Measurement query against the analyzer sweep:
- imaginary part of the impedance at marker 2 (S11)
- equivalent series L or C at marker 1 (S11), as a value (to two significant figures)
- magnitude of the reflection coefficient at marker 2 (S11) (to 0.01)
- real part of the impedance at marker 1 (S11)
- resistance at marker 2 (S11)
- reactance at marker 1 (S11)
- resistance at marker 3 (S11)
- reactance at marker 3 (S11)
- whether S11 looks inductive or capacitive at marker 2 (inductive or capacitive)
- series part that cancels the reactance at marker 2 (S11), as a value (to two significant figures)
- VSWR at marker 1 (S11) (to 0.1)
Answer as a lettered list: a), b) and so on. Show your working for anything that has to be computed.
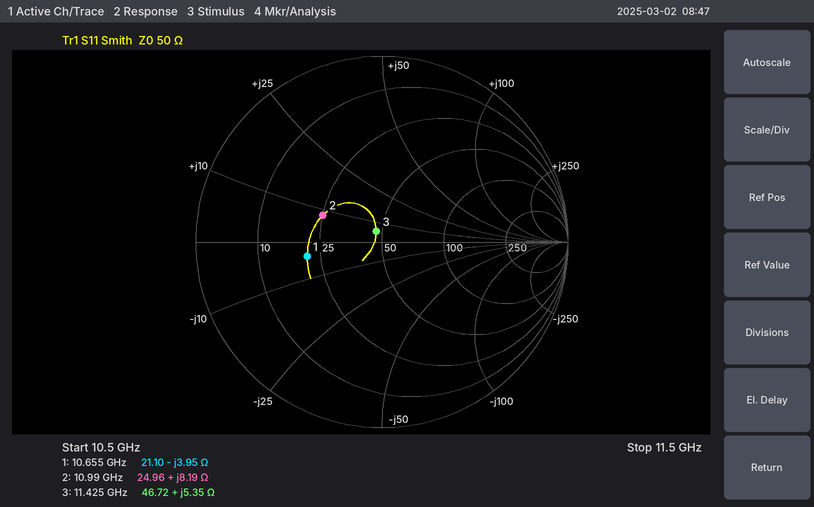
a) +8.19 Ω
b) C = 1/(2π × 10.655 GHz × 3.95 Ω) ≈ 3.8 pF
c) 0.35
d) 21.10 Ω
e) 24.96 Ω
f) -3.95 Ω
g) 46.72 Ω
h) +5.35 Ω
i) inductive
j) C = 1/(2π × 10.99 GHz × 8.19 Ω) ≈ 1.8 pF
k) 2.4
